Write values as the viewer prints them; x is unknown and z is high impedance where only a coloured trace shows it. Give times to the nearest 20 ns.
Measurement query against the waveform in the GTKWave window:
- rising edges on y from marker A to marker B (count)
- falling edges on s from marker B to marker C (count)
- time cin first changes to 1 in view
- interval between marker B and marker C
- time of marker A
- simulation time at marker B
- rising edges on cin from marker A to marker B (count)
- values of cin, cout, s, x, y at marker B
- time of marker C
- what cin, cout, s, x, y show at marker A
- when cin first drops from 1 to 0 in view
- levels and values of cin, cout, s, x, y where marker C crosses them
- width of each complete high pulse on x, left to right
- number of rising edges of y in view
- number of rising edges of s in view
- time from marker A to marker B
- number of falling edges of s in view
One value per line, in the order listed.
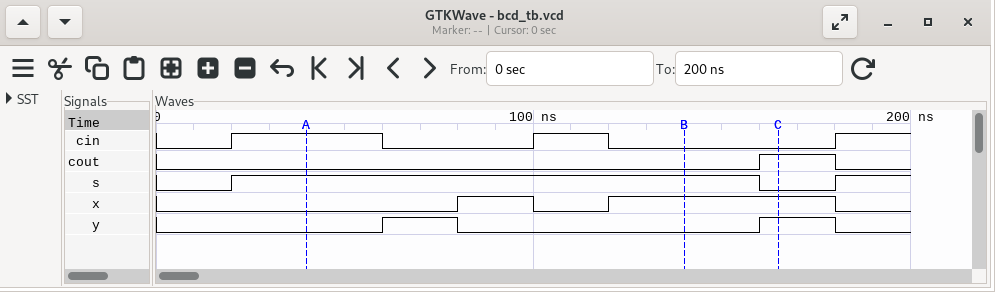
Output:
1
1
20 ns
20 ns
40 ns
140 ns
1
cin=0, cout=0, s=1, x=1, y=0
160 ns
cin=1, cout=0, s=1, x=0, y=0
60 ns
cin=0, cout=1, s=0, x=1, y=1
20 ns, 60 ns
2
2
100 ns
1
